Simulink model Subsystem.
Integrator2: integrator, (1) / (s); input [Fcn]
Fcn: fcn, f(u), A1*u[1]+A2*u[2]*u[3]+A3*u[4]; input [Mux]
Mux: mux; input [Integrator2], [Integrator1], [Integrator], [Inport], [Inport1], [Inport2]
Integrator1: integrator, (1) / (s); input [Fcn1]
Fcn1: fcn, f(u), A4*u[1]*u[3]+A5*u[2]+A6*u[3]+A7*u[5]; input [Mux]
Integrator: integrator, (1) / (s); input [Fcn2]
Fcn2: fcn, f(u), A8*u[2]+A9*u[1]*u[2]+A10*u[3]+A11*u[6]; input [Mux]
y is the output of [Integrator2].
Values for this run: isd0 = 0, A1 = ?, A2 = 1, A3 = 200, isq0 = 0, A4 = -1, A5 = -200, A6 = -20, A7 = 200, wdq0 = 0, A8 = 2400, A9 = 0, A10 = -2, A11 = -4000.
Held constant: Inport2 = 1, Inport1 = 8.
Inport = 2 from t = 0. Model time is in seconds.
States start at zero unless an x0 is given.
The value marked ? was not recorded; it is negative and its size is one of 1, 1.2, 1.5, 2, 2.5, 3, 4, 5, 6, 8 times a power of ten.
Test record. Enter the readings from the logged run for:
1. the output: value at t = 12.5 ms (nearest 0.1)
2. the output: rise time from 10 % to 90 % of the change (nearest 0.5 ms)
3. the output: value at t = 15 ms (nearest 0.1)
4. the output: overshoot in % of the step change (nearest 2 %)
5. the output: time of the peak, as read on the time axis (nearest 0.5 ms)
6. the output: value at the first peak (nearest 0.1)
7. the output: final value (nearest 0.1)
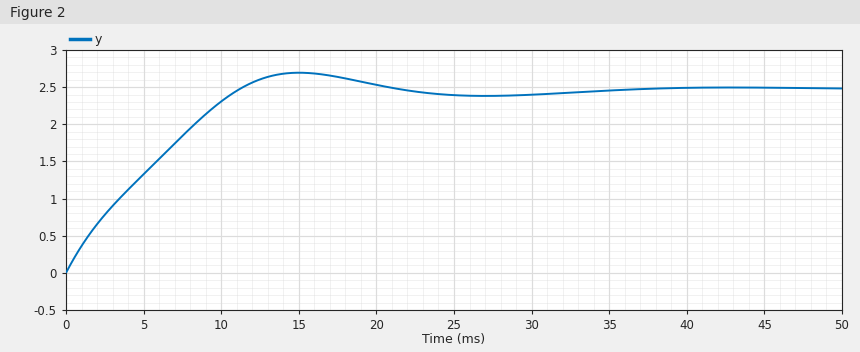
2.6
9.0 ms
2.7
8 %
15.0 ms
2.7
2.5
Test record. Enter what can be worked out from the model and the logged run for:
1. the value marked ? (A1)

-200
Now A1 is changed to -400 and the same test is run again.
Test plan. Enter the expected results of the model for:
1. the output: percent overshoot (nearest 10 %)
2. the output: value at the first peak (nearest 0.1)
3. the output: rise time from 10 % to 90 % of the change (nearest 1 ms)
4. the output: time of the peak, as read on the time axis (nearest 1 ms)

20 %
1.5
7 ms
13 ms
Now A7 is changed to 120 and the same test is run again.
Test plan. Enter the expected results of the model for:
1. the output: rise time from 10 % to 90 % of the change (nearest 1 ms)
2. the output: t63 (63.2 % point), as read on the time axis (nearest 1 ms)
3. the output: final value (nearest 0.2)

11 ms
6 ms
2.2
